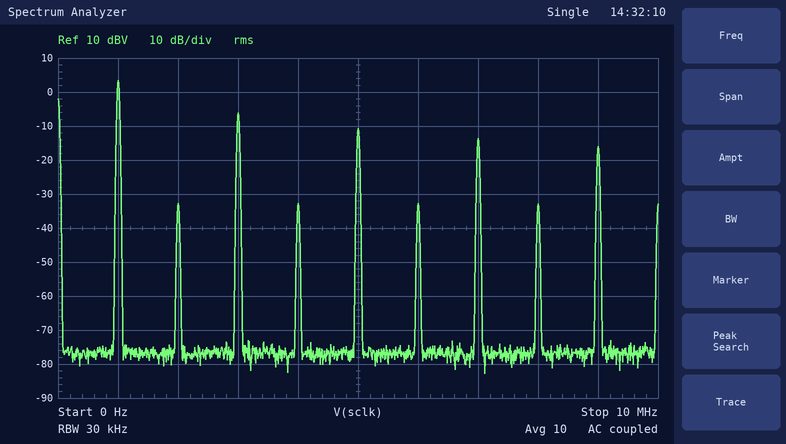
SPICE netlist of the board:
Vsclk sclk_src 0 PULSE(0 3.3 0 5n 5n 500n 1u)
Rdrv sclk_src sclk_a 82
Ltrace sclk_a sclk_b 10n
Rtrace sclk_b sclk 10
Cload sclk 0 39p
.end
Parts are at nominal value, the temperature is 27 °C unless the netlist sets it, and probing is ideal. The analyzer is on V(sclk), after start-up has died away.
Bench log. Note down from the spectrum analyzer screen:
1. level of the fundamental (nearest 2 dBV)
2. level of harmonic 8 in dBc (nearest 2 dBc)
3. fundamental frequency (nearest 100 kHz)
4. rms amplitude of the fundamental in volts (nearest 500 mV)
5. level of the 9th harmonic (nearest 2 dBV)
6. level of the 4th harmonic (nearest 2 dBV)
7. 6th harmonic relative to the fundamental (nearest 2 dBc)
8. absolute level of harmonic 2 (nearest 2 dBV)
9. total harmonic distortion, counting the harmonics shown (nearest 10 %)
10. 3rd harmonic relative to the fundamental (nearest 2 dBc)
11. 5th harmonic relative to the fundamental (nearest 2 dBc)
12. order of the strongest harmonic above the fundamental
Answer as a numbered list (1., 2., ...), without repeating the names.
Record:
1. 4 dBV
2. -36 dBc
3. 1.0 MHz
4. 1.5 V
5. -16 dBV
6. -32 dBV
7. -36 dBc
8. -32 dBV
9. 40 %
10. -10 dBc
11. -14 dBc
12. 3
